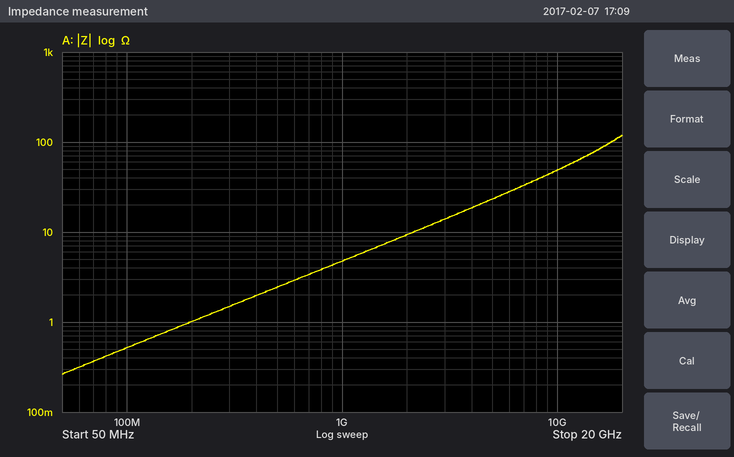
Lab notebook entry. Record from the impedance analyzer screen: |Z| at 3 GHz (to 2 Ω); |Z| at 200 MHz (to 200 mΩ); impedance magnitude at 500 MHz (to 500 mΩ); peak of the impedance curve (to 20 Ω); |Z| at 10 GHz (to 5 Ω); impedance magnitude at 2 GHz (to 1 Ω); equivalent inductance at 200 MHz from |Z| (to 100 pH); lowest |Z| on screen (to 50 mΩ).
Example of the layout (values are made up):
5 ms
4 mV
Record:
14 Ω
1.0 Ω
2.5 Ω
120 Ω
50 Ω
9 Ω
800 pH
250 mΩ
